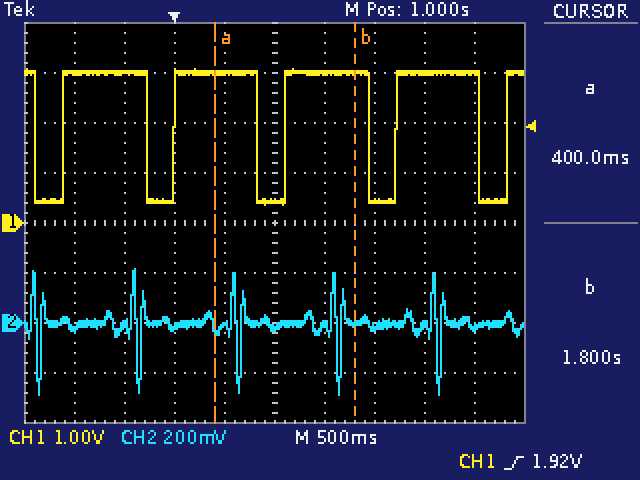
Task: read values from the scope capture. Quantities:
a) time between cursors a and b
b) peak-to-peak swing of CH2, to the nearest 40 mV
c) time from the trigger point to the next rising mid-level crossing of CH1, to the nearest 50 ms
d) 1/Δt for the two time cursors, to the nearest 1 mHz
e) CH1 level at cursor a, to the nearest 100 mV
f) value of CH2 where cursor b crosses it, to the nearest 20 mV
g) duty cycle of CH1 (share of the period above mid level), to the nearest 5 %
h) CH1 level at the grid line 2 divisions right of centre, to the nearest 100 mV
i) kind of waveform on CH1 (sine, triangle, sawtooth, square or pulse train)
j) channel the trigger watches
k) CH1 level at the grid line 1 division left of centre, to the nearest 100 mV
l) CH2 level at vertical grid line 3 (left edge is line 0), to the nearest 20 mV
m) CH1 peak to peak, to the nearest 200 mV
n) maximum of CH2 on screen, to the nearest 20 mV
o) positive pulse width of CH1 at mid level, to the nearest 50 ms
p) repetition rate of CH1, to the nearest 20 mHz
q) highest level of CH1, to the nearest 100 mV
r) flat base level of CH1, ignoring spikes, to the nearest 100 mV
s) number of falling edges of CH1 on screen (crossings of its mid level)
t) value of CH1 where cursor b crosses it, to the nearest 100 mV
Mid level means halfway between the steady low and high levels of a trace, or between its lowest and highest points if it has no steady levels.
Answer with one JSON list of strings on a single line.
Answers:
["1.40 s", "520 mV", "1.10 s", "714 mHz", "3.0 V", "0 mV", "75 %", "400 mV", "pulse train", "CH1", "3.0 V", "-20 mV", "2.8 V", "220 mV", "850 ms", "900 mHz", "3.1 V", "400 mV", "5", "3.0 V"]
